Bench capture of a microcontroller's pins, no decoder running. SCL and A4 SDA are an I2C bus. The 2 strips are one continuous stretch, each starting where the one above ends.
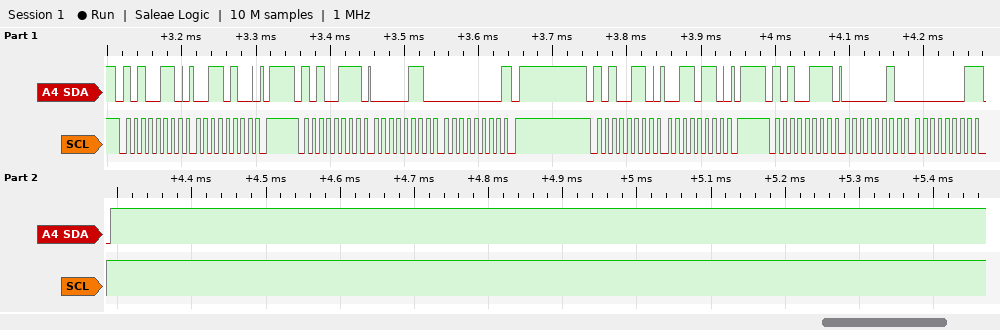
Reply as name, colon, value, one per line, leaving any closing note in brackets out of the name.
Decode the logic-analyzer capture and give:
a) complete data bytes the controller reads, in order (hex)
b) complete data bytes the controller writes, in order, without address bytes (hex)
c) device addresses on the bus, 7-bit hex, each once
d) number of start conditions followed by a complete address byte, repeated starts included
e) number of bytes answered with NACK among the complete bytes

complete data bytes the controller reads, in order: 06 00 02 01
complete data bytes the controller writes, in order, without address bytes: 34 36
device addresses on the bus, 7-bit hex, each once: 0x53
number of start conditions followed by a complete address byte, repeated starts included: 4
number of bytes answered with NACK among the complete bytes: 2
